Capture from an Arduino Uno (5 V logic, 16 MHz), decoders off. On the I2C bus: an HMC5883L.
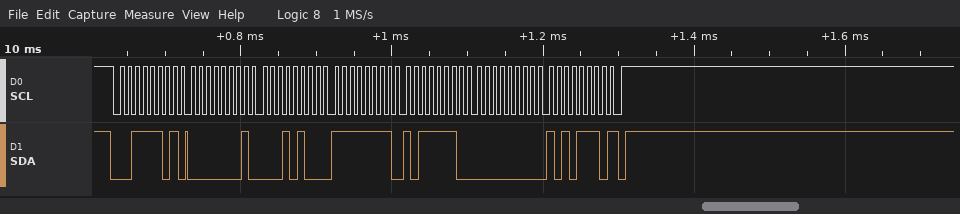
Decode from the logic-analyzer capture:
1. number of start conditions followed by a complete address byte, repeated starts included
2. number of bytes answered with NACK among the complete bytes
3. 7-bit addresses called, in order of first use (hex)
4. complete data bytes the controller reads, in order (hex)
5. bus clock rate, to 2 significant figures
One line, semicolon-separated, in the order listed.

1; 1; 0x1E; 01 14 FF BE 00 AE; 100 kHz
